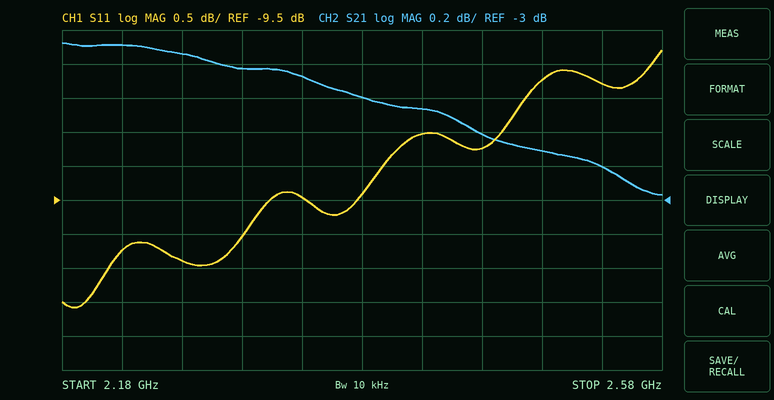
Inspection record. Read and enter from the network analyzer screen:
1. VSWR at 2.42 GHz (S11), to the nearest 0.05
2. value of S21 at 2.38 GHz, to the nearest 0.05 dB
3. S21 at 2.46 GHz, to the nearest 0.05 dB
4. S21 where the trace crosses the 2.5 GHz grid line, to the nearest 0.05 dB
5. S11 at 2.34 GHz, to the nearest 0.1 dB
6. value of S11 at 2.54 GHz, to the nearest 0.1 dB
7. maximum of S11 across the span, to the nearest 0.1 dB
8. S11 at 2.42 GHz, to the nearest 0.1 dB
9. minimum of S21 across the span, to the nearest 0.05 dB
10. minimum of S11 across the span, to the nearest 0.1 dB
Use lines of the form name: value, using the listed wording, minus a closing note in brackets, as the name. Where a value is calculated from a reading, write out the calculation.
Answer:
VSWR at 2.42 GHz (S11), to the nearest 0.05: |Γ| = 10^(-8.5/20) = 0.3758; VSWR = (1 + 0.3758)/(1 − 0.3758) ≈ 2.20
value of S21 at 2.38 GHz, to the nearest 0.05 dB: -2.40 dB
S21 at 2.46 GHz, to the nearest 0.05 dB: -2.60 dB
S21 where the trace crosses the 2.5 GHz grid line, to the nearest 0.05 dB: -2.70 dB
S11 at 2.34 GHz, to the nearest 0.1 dB: -9.5 dB
value of S11 at 2.54 GHz, to the nearest 0.1 dB: -7.8 dB
maximum of S11 across the span, to the nearest 0.1 dB: -7.3 dB
S11 at 2.42 GHz, to the nearest 0.1 dB: -8.5 dB
minimum of S21 across the span, to the nearest 0.05 dB: -2.95 dB
minimum of S11 across the span, to the nearest 0.1 dB: -11.1 dB
